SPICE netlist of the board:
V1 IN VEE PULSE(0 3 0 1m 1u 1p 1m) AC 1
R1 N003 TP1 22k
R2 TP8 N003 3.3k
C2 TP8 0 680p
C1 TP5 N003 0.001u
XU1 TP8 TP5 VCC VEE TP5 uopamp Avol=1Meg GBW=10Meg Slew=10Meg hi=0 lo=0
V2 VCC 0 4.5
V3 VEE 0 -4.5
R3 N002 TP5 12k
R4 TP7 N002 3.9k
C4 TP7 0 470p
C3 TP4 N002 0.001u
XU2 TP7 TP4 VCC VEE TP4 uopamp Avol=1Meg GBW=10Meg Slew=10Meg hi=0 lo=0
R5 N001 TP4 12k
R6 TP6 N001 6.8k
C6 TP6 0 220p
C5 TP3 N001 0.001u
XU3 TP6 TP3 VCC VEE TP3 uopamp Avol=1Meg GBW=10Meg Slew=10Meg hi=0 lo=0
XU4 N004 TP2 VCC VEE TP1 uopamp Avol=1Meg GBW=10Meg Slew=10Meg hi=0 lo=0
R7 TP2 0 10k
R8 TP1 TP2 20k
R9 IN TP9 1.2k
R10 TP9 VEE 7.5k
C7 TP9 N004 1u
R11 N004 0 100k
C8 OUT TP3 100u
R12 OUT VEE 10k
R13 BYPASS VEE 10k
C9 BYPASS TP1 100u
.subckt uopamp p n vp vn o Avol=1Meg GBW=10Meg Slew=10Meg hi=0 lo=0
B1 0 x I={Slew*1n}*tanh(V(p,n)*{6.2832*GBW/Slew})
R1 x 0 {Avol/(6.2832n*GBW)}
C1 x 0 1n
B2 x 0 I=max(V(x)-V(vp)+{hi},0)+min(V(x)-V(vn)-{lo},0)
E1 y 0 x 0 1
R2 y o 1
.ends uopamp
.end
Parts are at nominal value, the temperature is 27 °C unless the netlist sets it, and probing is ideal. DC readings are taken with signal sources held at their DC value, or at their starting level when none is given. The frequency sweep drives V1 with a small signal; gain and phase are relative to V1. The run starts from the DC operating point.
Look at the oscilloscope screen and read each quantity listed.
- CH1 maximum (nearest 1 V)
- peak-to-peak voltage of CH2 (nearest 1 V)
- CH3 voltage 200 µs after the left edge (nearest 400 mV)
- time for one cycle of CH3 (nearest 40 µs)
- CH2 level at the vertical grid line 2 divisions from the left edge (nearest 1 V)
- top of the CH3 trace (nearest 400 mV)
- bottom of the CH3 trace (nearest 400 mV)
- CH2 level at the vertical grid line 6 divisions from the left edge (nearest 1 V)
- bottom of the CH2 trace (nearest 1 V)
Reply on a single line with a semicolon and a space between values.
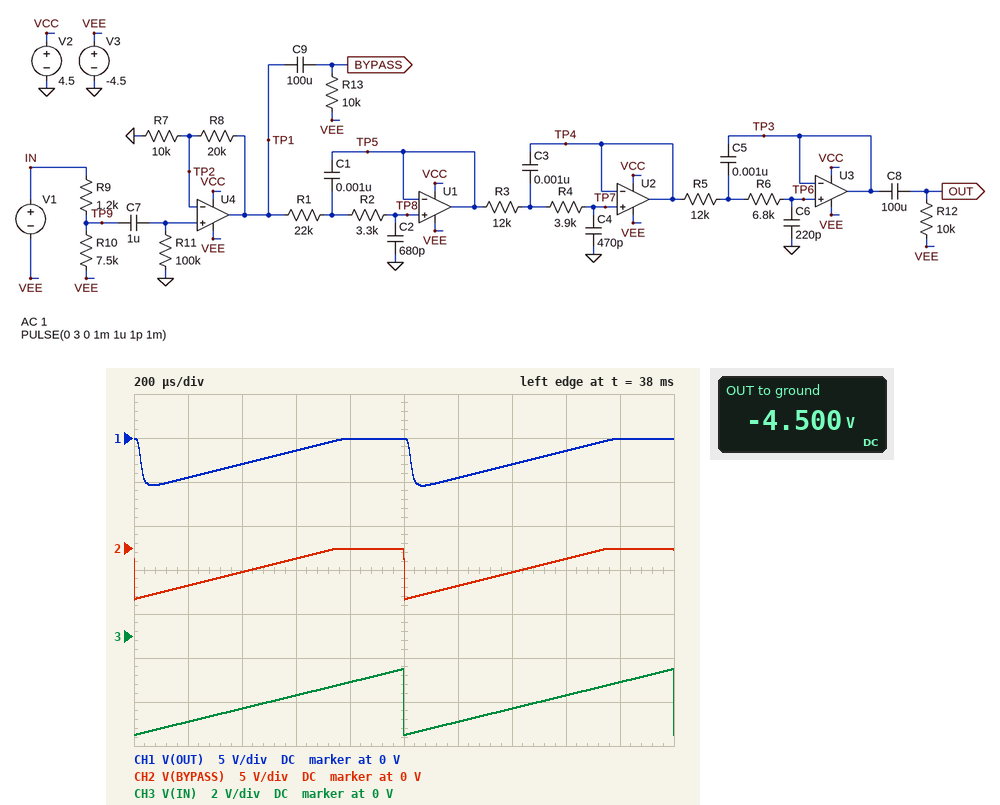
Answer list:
0 V; 6 V; -4.0 V; 1.00 ms; -3 V; -1.6 V; -4.4 V; -4 V; -6 V
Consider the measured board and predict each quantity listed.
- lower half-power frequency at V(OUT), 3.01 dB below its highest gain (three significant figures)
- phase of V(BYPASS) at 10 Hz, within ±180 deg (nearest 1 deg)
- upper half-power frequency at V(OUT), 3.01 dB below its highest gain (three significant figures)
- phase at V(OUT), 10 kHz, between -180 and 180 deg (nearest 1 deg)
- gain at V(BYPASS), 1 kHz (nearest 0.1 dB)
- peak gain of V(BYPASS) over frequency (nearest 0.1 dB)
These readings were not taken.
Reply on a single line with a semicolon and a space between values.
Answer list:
1.59 Hz; 10 deg; 11.3 kHz; -97 deg; 8.2 dB; 8.2 dB
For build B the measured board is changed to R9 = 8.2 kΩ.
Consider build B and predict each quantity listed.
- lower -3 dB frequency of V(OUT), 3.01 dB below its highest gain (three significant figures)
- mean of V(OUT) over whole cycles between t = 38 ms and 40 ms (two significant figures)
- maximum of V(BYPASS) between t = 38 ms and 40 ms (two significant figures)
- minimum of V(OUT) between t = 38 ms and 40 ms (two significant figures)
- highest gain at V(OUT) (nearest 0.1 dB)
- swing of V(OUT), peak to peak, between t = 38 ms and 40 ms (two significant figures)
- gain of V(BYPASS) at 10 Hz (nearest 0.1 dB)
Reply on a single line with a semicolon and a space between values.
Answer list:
1.55 Hz; -3.1 V; -1.1 V; -5.0 V; 2.8 dB; 3.8 V; 2.7 dB
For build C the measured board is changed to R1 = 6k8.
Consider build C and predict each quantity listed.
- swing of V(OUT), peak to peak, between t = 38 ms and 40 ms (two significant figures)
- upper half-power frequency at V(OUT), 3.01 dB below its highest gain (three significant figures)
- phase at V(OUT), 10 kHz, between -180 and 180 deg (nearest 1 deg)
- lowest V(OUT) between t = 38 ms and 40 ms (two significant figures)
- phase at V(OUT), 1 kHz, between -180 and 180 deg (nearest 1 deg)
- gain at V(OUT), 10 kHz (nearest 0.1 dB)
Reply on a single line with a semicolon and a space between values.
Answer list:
6.0 V; 26.5 kHz; -68 deg; -6.1 V; -7 deg; 8.0 dB
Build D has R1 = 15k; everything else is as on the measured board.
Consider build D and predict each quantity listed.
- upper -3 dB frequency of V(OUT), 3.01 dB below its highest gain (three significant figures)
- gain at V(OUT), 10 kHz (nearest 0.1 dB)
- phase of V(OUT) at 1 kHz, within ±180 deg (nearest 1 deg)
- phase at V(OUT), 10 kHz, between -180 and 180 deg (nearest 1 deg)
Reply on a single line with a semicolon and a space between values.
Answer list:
16.3 kHz; 6.9 dB; -9 deg; -85 deg
